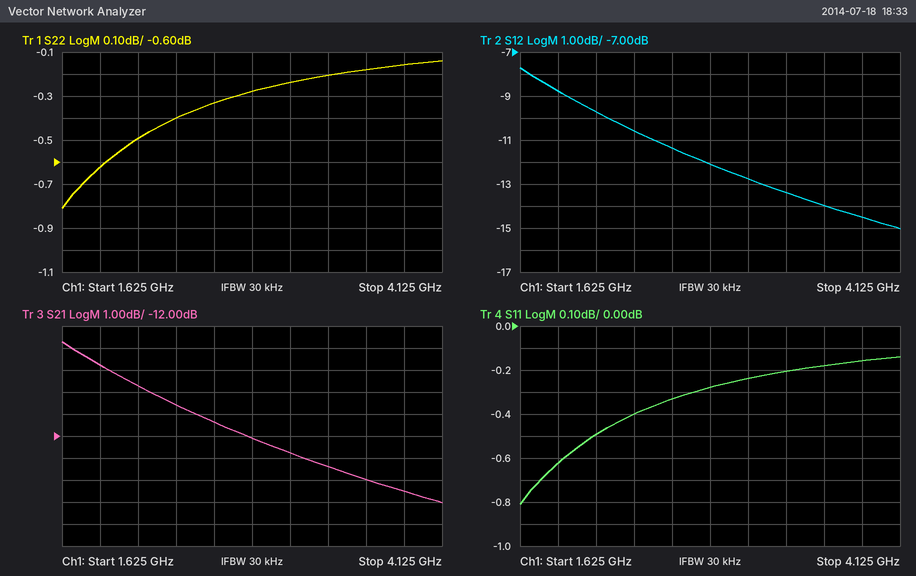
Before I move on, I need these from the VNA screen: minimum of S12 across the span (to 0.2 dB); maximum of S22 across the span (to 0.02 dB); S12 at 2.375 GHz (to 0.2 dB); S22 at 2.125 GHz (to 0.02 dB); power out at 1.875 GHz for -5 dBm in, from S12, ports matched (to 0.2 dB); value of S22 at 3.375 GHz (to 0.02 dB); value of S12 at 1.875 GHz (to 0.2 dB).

-15.0 dB
-0.14 dB
-10.6 dB
-0.50 dB
-13.8 dBm
-0.20 dB
-8.8 dB
